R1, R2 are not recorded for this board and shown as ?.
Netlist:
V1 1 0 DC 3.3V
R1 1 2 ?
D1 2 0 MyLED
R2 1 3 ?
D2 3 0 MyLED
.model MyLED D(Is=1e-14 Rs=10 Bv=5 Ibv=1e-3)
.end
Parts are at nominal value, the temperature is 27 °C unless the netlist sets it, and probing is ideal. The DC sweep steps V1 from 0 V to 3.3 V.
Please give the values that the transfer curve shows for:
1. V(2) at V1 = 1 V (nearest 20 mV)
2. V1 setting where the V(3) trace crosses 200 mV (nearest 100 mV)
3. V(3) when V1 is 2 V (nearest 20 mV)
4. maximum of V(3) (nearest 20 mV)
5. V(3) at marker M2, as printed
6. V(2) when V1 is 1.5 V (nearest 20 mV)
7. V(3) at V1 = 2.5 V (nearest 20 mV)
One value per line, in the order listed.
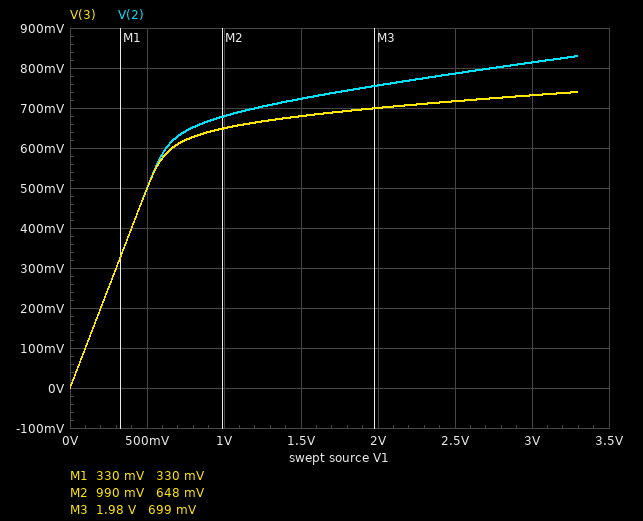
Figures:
680 mV
200 mV
700 mV
740 mV
648 mV
720 mV
720 mV
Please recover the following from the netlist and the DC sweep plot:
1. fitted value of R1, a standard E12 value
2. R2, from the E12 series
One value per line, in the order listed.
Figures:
220 Ω
560 Ω
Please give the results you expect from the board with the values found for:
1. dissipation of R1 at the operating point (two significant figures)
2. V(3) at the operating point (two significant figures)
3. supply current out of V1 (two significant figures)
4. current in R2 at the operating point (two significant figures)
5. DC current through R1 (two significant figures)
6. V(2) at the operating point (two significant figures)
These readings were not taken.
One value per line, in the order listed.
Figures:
28 mW
740 mV
16 mA
4.6 mA
11 mA
830 mV
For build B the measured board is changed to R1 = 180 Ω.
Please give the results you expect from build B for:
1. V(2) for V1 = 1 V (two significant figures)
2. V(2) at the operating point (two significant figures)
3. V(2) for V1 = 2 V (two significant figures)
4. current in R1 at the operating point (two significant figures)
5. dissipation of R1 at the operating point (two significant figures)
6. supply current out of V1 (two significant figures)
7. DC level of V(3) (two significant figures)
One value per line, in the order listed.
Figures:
690 mV
860 mV
770 mV
14 mA
33 mW
18 mA
740 mV
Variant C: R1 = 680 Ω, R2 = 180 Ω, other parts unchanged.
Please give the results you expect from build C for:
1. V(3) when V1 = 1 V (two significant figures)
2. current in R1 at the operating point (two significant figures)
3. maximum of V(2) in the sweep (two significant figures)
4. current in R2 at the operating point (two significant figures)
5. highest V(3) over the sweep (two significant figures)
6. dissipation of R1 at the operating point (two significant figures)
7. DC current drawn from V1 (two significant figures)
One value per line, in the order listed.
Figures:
690 mV
3.8 mA
730 mV
14 mA
860 mV
9.7 mW
17 mA
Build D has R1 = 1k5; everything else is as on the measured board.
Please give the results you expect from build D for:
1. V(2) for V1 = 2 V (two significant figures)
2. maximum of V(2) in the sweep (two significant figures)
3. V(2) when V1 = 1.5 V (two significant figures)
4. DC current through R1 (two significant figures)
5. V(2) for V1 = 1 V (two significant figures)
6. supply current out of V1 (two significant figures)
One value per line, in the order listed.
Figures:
660 mV
690 mV
650 mV
1.7 mA
620 mV
6.3 mA
